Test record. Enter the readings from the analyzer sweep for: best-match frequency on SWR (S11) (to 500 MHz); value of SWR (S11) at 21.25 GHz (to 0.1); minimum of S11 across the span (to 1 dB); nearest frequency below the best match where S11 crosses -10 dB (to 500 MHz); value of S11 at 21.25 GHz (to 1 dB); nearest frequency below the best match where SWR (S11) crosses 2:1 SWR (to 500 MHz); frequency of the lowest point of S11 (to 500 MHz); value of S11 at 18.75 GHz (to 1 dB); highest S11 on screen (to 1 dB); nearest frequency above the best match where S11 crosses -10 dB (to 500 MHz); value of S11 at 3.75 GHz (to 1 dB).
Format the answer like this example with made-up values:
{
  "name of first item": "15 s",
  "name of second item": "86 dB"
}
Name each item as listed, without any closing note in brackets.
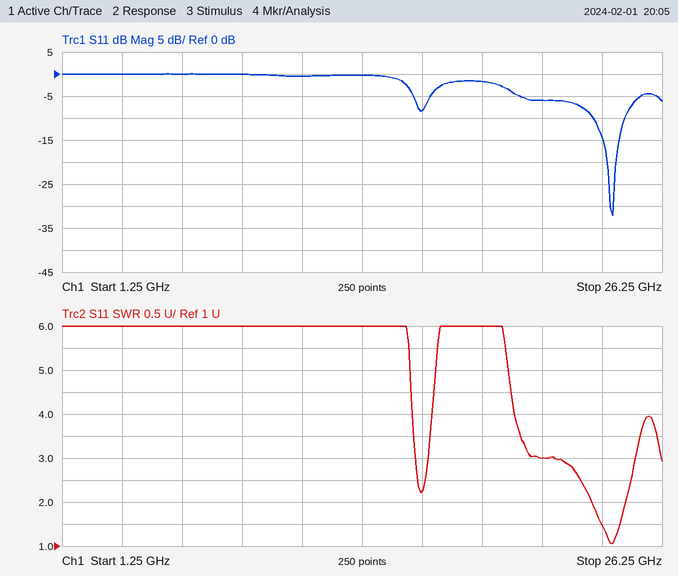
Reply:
{
  "best-match frequency on SWR (S11)": "24.0 GHz",
  "value of SWR (S11) at 21.25 GHz": "3.0",
  "minimum of S11 across the span": "-32 dB",
  "nearest frequency below the best match where S11 crosses -10 dB": "23.5 GHz",
  "value of S11 at 21.25 GHz": "-6 dB",
  "nearest frequency below the best match where SWR (S11) crosses 2:1 SWR": "23.5 GHz",
  "frequency of the lowest point of S11": "24.0 GHz",
  "value of S11 at 18.75 GHz": "-2 dB",
  "highest S11 on screen": "0 dB",
  "nearest frequency above the best match where S11 crosses -10 dB": "24.5 GHz",
  "value of S11 at 3.75 GHz": "0 dB"
}
